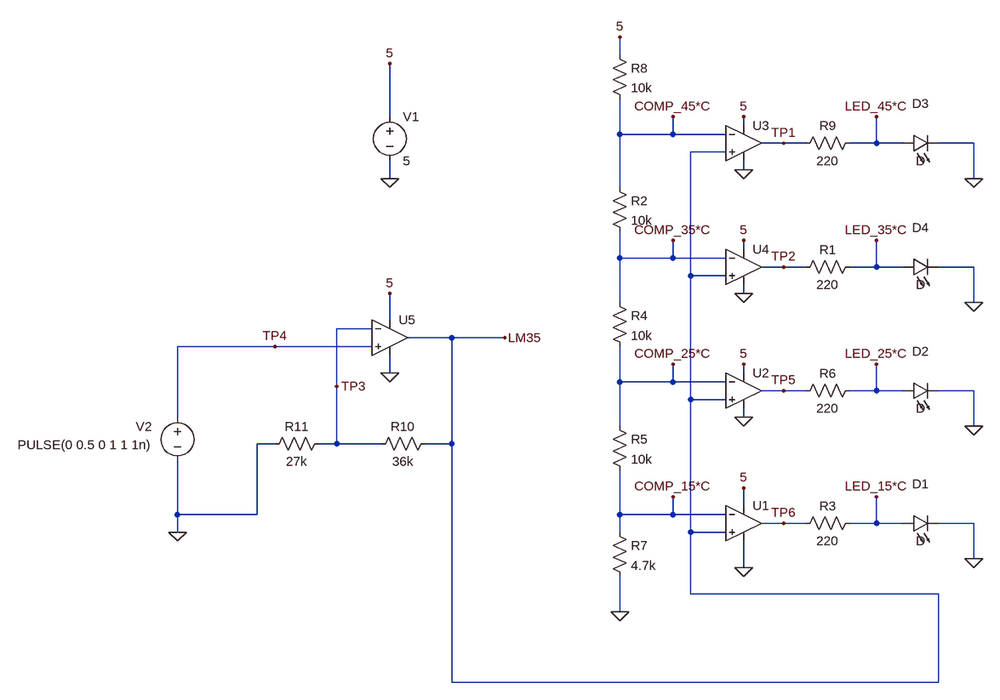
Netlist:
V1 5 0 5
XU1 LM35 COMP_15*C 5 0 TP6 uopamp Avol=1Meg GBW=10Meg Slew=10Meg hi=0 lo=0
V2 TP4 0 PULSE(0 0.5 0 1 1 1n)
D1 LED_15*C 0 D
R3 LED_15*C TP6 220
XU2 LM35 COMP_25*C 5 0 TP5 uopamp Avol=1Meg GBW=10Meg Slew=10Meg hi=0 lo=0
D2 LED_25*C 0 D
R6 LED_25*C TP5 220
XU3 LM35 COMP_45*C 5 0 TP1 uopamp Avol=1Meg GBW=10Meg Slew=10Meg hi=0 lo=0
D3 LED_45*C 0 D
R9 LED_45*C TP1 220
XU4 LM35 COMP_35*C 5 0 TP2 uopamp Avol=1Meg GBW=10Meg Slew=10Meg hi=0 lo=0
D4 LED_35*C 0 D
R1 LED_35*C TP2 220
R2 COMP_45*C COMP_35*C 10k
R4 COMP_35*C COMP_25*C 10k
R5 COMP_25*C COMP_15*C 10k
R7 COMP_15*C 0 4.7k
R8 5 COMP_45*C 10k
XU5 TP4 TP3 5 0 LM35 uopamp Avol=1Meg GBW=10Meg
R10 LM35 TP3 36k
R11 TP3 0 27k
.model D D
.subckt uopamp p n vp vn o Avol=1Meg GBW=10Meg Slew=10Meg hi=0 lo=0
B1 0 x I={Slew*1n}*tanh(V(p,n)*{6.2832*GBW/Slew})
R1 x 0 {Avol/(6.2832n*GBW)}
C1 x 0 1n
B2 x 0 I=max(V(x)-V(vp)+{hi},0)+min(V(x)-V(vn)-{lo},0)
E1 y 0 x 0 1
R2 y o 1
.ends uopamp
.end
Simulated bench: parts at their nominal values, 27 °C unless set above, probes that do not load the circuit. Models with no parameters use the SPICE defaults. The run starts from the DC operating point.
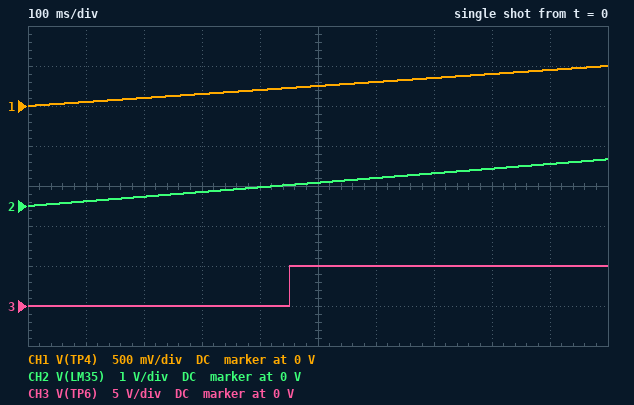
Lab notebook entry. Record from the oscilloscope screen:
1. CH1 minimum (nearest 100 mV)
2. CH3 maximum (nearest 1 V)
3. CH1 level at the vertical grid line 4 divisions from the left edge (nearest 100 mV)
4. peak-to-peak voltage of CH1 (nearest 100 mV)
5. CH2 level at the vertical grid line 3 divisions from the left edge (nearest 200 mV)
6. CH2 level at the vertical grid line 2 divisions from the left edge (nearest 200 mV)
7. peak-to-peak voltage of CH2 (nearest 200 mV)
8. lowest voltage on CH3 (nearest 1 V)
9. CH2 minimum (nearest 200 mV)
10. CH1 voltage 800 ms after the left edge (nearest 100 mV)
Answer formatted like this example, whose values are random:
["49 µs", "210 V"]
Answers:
["0 V", "5 V", "200 mV", "500 mV", "400 mV", "200 mV", "1.2 V", "0 V", "0 V", "400 mV"]
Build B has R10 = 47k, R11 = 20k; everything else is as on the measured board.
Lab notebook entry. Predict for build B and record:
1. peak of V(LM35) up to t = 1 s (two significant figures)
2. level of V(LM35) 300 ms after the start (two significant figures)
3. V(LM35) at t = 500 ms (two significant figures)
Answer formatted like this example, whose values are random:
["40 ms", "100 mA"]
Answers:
["1.7 V", "500 mV", "840 mV"]
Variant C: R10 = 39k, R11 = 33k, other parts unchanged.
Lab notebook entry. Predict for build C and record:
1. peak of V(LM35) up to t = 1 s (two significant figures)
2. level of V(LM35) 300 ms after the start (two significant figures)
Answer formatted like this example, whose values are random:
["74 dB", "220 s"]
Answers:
["1.1 V", "330 mV"]
